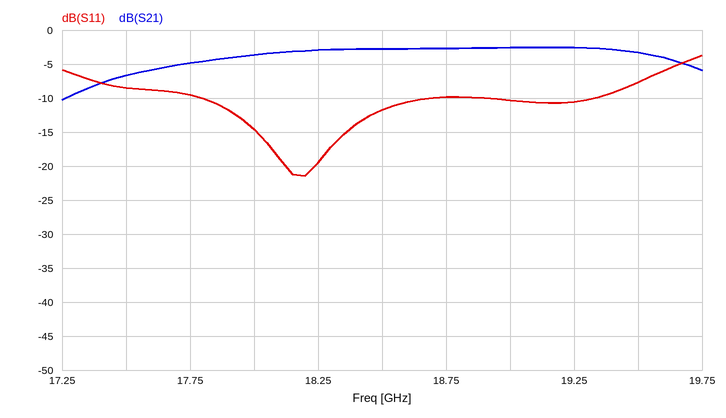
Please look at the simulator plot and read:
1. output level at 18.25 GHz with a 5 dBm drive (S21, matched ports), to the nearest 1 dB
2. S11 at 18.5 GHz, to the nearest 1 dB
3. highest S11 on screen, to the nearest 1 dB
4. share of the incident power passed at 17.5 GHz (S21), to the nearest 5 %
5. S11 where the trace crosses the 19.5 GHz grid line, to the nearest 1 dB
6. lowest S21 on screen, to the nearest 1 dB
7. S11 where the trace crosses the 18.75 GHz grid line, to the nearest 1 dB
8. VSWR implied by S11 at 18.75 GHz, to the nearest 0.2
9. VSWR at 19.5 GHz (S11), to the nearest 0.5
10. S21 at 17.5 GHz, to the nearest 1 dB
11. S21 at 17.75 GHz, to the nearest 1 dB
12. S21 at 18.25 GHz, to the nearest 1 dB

2 dBm
-12 dB
-4 dB
20 %
-8 dB
-10 dB
-10 dB
2.0
2.5
-7 dB
-5 dB
-3 dB
